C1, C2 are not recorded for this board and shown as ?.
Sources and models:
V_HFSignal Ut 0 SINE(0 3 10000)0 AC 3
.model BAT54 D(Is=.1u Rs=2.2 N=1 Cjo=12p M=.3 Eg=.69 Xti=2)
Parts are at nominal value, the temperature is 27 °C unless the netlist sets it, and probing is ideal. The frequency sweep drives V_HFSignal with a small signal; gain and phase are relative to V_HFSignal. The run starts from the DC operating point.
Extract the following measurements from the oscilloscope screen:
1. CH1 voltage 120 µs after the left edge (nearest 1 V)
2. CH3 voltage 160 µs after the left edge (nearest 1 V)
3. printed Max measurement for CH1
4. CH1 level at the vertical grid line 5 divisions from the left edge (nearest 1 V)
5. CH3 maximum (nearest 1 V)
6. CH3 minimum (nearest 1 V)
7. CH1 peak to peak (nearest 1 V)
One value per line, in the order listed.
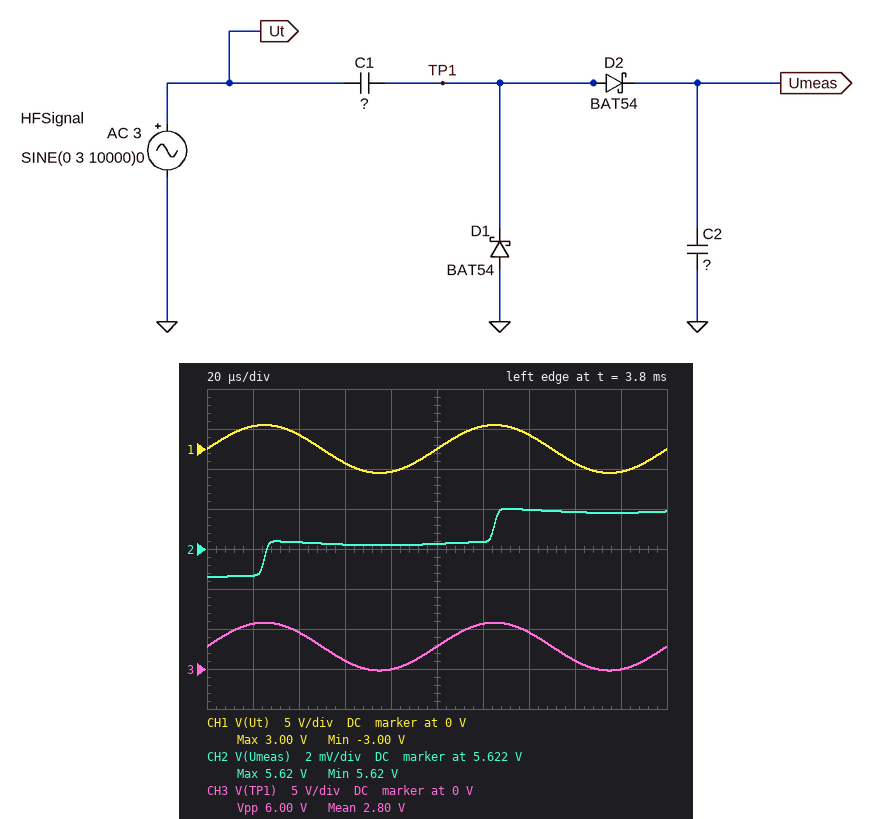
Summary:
3 V
1 V
3.00 V
0 V
6 V
0 V
6 V
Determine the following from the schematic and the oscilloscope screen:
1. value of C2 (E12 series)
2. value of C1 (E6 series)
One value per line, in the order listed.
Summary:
270 nF
220 nF
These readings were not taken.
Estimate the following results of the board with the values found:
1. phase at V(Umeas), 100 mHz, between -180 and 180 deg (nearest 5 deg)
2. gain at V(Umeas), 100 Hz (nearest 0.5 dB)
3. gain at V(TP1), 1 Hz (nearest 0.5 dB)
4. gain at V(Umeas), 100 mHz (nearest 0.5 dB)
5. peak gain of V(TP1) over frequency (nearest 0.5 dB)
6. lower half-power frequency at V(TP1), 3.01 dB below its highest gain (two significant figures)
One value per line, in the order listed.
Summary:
85 deg
-33.0 dB
-11.5 dB
-29.0 dB
0 dB
6.3 Hz
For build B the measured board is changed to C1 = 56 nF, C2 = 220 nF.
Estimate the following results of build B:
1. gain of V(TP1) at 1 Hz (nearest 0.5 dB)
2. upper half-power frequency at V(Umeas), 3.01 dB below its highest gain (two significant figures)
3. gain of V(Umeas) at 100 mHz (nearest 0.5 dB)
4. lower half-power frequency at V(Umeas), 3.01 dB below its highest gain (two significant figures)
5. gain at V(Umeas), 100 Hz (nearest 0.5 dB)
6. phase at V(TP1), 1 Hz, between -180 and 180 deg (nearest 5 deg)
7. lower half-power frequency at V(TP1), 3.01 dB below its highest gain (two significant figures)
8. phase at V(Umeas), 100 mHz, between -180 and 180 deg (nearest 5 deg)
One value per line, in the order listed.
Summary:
-22.5 dB
26 Hz
-41.0 dB
1.2 Hz
-31.5 dB
70 deg
23 Hz
85 deg
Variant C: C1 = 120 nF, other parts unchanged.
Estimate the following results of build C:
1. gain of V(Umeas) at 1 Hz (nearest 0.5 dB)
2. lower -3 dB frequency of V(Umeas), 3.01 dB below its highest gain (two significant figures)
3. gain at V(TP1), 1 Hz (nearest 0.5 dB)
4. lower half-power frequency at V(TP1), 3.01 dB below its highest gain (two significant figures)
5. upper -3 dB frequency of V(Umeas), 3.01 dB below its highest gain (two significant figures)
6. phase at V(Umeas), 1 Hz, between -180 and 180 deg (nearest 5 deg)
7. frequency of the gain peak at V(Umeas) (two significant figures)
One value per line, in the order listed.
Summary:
-17.0 dB
870 mHz
-16.5 dB
11 Hz
13 Hz
40 deg
3.4 Hz
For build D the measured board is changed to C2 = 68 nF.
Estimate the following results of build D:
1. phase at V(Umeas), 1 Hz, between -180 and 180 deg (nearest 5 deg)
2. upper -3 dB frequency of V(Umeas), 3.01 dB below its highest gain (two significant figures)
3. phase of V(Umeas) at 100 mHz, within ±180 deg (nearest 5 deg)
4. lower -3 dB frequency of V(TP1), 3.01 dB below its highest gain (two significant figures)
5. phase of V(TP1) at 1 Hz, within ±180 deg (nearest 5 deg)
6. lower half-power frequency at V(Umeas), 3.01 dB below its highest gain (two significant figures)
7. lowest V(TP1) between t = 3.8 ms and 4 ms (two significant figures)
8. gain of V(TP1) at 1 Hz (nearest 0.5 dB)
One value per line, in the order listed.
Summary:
60 deg
16 Hz
85 deg
5.0 Hz
65 deg
1.6 Hz
-170 mV
-10.0 dB
